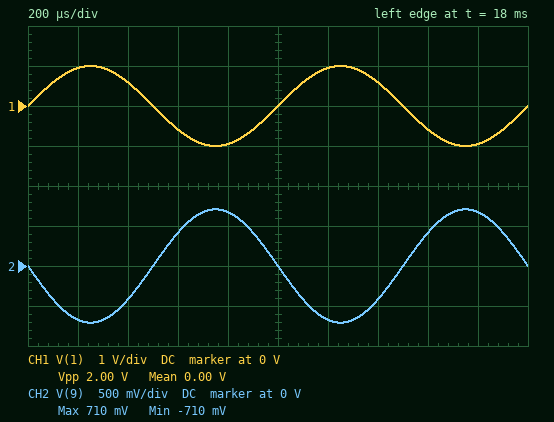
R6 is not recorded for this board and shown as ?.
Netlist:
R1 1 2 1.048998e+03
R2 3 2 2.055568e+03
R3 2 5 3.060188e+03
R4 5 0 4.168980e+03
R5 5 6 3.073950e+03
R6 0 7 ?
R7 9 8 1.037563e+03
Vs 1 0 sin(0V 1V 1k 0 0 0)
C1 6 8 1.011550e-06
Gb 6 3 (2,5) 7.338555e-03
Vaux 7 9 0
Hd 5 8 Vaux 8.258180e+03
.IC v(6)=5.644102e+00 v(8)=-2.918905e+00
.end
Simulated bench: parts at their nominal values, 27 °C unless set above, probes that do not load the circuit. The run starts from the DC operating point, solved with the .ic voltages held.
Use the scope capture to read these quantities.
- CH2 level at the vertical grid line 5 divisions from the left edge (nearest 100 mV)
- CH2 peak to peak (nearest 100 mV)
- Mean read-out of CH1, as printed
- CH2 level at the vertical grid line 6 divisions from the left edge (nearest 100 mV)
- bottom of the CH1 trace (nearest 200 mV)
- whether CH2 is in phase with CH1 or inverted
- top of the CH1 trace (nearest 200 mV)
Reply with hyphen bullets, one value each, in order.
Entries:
- 0 V
- 1.4 V
- 0.00 V
- -700 mV
- -1.0 V
- inverted
- 1.0 V
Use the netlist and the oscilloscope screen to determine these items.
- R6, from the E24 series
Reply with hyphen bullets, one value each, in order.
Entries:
- 3 kΩ
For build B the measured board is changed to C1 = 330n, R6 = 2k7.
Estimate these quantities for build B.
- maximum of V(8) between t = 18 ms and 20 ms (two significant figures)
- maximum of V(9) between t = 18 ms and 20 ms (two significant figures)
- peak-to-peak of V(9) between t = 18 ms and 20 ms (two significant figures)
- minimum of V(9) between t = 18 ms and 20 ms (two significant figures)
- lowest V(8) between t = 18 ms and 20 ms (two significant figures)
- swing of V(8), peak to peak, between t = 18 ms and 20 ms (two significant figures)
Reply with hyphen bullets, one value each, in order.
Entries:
- 810 mV
- 590 mV
- 1.2 V
- -590 mV
- -810 mV
- 1.6 V
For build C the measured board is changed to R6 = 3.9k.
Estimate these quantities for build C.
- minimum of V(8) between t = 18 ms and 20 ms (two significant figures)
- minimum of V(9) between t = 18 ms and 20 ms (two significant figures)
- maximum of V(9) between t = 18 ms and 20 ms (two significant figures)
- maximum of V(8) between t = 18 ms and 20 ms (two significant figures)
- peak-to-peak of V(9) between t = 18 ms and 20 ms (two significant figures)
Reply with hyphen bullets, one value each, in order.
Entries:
- -1.6 V
- -1.2 V
- 1.2 V
- 1.6 V
- 2.5 V
